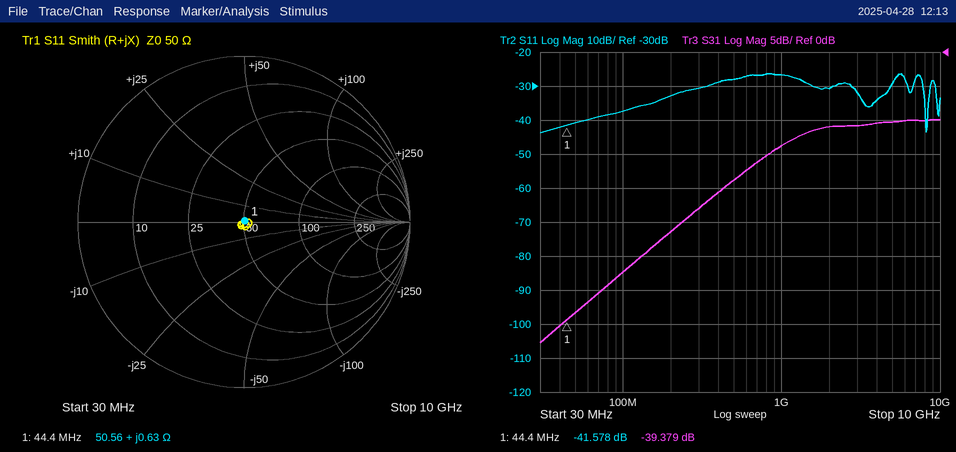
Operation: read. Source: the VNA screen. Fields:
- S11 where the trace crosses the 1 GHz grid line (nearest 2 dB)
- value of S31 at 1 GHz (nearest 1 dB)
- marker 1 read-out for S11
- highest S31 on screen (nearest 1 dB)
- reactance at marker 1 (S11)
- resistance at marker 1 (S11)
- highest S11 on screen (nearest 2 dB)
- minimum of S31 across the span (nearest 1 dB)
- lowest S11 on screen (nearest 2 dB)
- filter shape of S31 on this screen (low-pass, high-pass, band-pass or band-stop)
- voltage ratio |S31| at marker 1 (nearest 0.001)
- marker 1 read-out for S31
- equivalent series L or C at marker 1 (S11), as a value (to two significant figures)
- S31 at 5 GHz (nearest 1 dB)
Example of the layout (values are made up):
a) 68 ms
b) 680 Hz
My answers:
a) -26 dB
b) -14 dB
c) -41.578 dB
d) -10 dB
e) +0.63 Ω
f) 50.56 Ω
g) -26 dB
h) -43 dB
i) -44 dB
j) high-pass
k) 0.011
l) -39.379 dB
m) 2.3 nH
n) -10 dB
